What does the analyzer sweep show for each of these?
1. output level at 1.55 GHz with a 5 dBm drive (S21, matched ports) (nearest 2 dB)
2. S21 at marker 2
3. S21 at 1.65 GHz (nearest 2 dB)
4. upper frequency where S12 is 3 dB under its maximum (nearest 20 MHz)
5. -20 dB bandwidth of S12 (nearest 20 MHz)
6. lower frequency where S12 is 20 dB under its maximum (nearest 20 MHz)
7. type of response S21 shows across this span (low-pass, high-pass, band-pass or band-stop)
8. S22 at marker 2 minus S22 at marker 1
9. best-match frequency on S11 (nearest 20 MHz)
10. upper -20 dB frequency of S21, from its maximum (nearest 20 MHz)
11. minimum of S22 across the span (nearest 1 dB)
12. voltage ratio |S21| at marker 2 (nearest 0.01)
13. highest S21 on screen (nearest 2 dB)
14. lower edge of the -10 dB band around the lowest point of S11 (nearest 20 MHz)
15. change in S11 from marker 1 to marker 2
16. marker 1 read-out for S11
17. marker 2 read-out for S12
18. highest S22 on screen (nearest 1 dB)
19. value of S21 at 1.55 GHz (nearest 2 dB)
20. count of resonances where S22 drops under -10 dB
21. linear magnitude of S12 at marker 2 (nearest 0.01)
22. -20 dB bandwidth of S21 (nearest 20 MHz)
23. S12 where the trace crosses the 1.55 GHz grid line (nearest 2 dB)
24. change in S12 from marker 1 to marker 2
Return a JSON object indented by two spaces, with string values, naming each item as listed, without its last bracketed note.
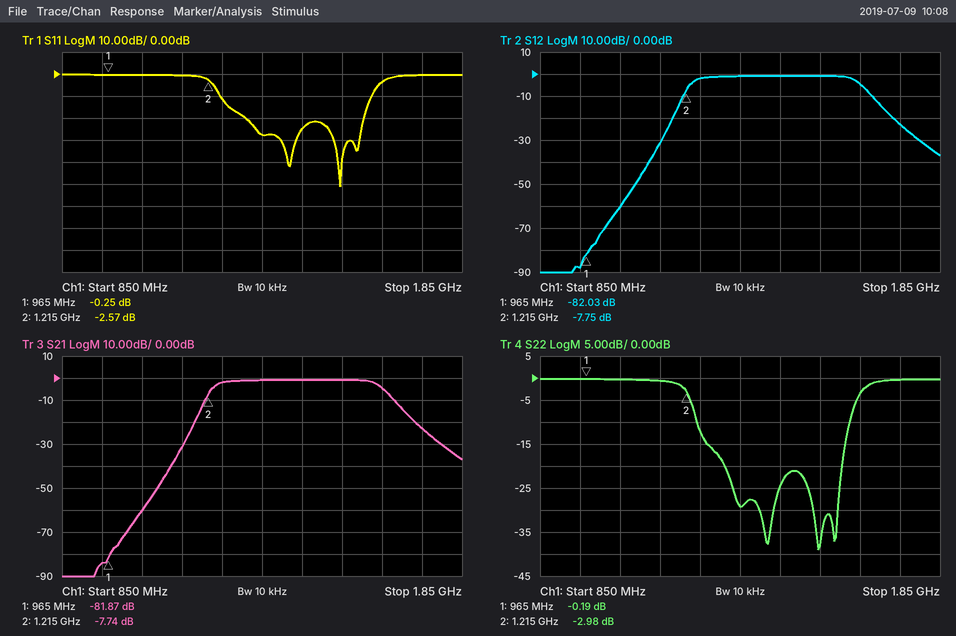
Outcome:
{
  "output level at 1.55 GHz with a 5 dBm drive (S21, matched ports)": "4 dBm",
  "S21 at marker 2": "-7.74 dB",
  "S21 at 1.65 GHz": "-4 dB",
  "upper frequency where S12 is 3 dB under its maximum": "1.64 GHz",
  "-20 dB bandwidth of S12": "560 MHz",
  "lower frequency where S12 is 20 dB under its maximum": "1.18 GHz",
  "type of response S21 shows across this span": "band-pass",
  "S22 at marker 2 minus S22 at marker 1": "-2.79 dB",
  "best-match frequency on S11": "1.54 GHz",
  "upper -20 dB frequency of S21, from its maximum": "1.74 GHz",
  "minimum of S22 across the span": "-39 dB",
  "voltage ratio |S21| at marker 2": "0.41",
  "highest S21 on screen": "0 dB",
  "lower edge of the -10 dB band around the lowest point of S11": "1.24 GHz",
  "change in S11 from marker 1 to marker 2": "-2.32 dB",
  "marker 1 read-out for S11": "-0.25 dB",
  "marker 2 read-out for S12": "-7.75 dB",
  "highest S22 on screen": "0 dB",
  "value of S21 at 1.55 GHz": "0 dB",
  "count of resonances where S22 drops under -10 dB": "3",
  "linear magnitude of S12 at marker 2": "0.41",
  "-20 dB bandwidth of S21": "560 MHz",
  "S12 where the trace crosses the 1.55 GHz grid line": "0 dB",
  "change in S12 from marker 1 to marker 2": "74.28 dB"
}
